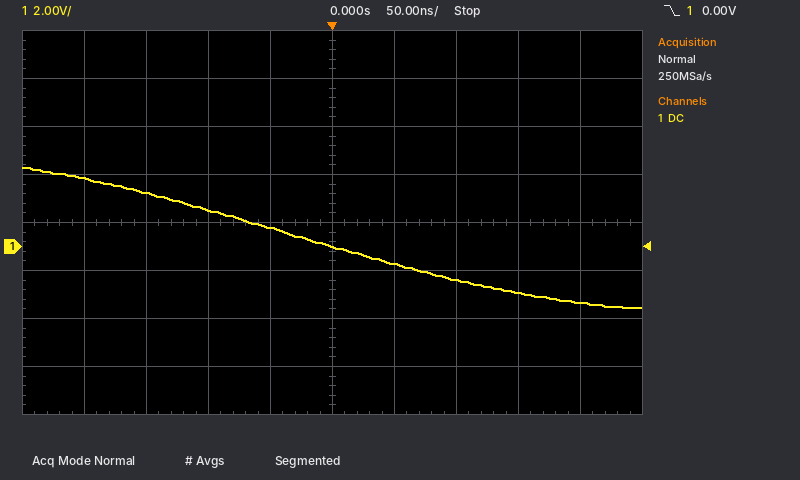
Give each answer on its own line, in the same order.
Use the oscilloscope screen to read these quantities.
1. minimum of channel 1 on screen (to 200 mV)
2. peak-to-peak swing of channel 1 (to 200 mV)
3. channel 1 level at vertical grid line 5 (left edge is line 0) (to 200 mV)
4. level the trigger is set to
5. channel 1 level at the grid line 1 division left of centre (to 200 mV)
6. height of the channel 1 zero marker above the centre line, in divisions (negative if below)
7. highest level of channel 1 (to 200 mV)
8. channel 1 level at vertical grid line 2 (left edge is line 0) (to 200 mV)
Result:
-2.6 V
5.8 V
0.0 V
0.00 V
800 mV
-0.5 div
3.2 V
2.2 V
